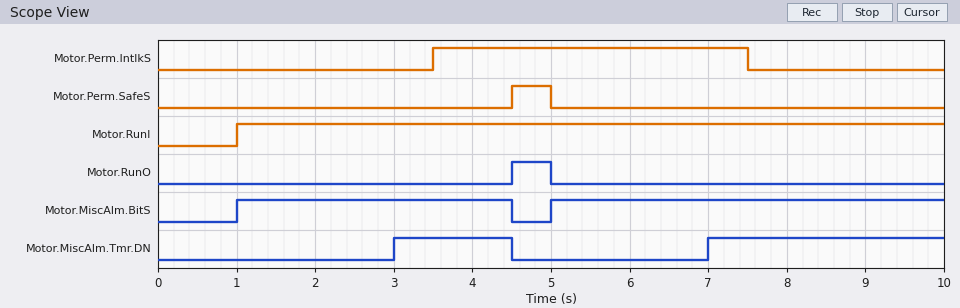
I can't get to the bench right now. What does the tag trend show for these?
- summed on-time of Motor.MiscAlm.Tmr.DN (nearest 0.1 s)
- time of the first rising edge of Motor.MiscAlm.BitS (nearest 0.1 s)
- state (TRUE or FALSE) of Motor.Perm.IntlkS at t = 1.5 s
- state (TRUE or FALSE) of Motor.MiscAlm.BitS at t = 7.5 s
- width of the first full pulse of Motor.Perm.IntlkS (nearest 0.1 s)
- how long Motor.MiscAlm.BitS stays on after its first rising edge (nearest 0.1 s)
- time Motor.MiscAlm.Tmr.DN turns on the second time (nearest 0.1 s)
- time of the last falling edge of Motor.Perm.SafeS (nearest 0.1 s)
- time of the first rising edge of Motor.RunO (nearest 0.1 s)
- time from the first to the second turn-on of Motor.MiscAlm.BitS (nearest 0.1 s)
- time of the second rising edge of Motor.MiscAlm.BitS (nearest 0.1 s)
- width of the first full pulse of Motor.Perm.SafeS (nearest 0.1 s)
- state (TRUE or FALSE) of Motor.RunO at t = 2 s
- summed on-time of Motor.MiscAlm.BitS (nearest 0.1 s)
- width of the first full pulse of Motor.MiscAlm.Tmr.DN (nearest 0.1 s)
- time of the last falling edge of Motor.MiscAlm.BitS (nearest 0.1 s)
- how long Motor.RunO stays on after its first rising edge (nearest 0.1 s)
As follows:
4.5 s
1.0 s
FALSE
TRUE
4.0 s
3.5 s
7.0 s
5.0 s
4.5 s
4.0 s
5.0 s
0.5 s
FALSE
8.5 s
1.5 s
4.5 s
0.5 s
